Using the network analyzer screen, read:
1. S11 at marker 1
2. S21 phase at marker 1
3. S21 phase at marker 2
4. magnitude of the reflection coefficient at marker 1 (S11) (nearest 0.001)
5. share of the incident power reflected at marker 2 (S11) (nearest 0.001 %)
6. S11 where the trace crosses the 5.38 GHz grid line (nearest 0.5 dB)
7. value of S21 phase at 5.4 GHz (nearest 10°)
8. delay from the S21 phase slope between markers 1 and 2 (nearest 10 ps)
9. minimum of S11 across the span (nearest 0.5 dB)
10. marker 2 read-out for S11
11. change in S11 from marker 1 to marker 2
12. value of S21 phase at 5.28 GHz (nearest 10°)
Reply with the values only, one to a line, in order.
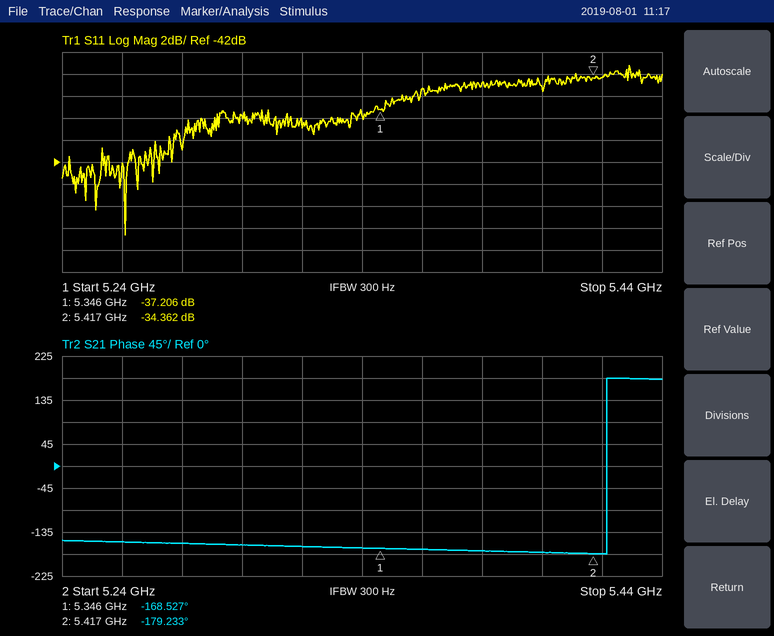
-37.206 dB
-168.527°
-179.233°
0.014
0.037 %
-35.0 dB
-180°
420 ps
-48.5 dB
-34.362 dB
2.844 dB
-160°
